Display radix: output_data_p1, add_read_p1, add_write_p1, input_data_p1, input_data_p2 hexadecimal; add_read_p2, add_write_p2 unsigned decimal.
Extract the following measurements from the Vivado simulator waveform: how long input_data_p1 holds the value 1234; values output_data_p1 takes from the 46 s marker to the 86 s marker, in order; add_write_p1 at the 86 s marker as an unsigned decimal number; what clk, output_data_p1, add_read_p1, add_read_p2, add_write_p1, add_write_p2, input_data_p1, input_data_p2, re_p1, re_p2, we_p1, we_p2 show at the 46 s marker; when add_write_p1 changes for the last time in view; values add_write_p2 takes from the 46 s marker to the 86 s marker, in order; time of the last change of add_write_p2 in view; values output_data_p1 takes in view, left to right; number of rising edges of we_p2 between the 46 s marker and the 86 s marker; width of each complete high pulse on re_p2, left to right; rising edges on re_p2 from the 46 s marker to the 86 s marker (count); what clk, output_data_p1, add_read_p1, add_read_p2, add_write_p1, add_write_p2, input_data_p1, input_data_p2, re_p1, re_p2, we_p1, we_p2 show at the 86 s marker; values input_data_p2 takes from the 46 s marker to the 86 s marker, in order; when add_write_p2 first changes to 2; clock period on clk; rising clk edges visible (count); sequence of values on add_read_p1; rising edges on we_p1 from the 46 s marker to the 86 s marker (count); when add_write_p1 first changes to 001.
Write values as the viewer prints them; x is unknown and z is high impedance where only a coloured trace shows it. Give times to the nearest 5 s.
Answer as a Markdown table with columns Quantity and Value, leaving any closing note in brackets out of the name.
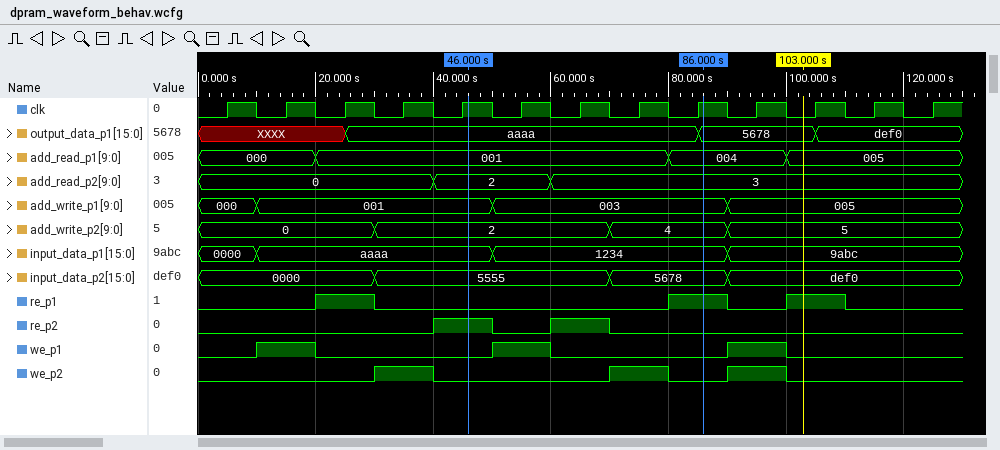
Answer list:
| Quantity | Value |
|---|---|
| how long input_data_p1 holds the value 1234 | 40 s |
| values output_data_p1 takes from the 46 s marker to the 86 s marker, in order | aaaa, 5678 |
| add_write_p1 at the 86 s marker as an unsigned decimal number | 3 |
| what clk, output_data_p1, add_read_p1, add_read_p2, add_write_p1, add_write_p2, input_data_p1, input_data_p2, re_p1, re_p2, we_p1, we_p2 show at the 46 s marker | clk=1, output_data_p1=aaaa, add_read_p1=001, add_read_p2=2, add_write_p1=001, add_write_p2=2, input_data_p1=aaaa, input_data_p2=5555, re_p1=0, re_p2=1, we_p1=0, we_p2=0 |
| when add_write_p1 changes for the last time in view | 90 s |
| values add_write_p2 takes from the 46 s marker to the 86 s marker, in order | 2, 4 |
| time of the last change of add_write_p2 in view | 90 s |
| values output_data_p1 takes in view, left to right | XXXX, aaaa, 5678, def0 |
| number of rising edges of we_p2 between the 46 s marker and the 86 s marker | 1 |
| width of each complete high pulse on re_p2, left to right | 10 s, 10 s |
| rising edges on re_p2 from the 46 s marker to the 86 s marker | 1 |
| what clk, output_data_p1, add_read_p1, add_read_p2, add_write_p1, add_write_p2, input_data_p1, input_data_p2, re_p1, re_p2, we_p1, we_p2 show at the 86 s marker | clk=1, output_data_p1=5678, add_read_p1=004, add_read_p2=3, add_write_p1=003, add_write_p2=4, input_data_p1=1234, input_data_p2=5678, re_p1=1, re_p2=0, we_p1=0, we_p2=0 |
| values input_data_p2 takes from the 46 s marker to the 86 s marker, in order | 5555, 5678 |
| when add_write_p2 first changes to 2 | 30 s |
| clock period on clk | 10 s |
| rising clk edges visible | 13 |
| sequence of values on add_read_p1 | 000, 001, 004, 005 |
| rising edges on we_p1 from the 46 s marker to the 86 s marker | 1 |
| when add_write_p1 first changes to 001 | 10 s |
